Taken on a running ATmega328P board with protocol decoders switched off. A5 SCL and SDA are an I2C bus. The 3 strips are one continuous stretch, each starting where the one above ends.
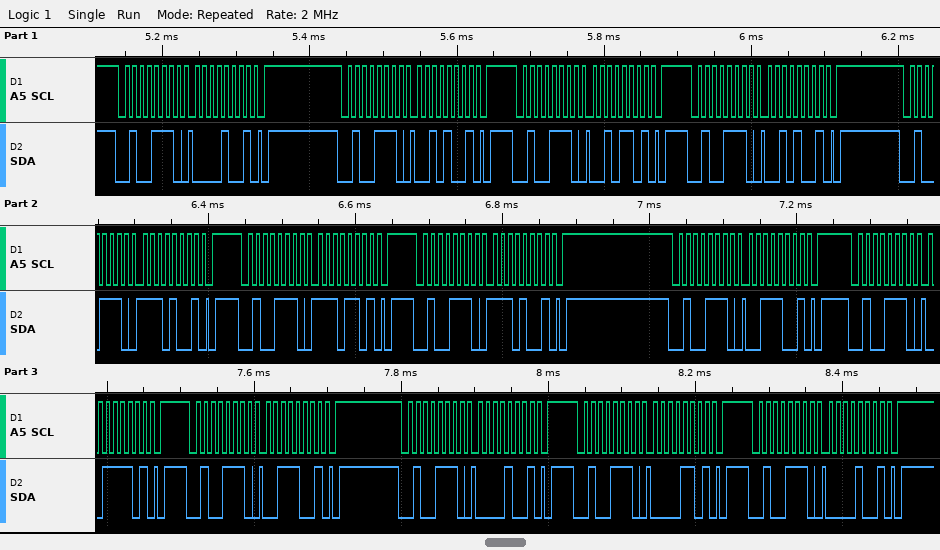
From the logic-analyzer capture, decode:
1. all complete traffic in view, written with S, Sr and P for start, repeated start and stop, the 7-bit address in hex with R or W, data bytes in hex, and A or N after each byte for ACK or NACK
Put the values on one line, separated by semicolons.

S 27W A 09 A P S 27W A 29 A P S 27W A 2D A P S 27W A 29 A P S 27W A E9 A P S 27W A ED A P S 27W A E9 A P S 27W A 39 A P S 27W A 3D A P S 27W A 39 A P S 27W A 09 A P S 27W A 0D A P S 27W A 09 A P
